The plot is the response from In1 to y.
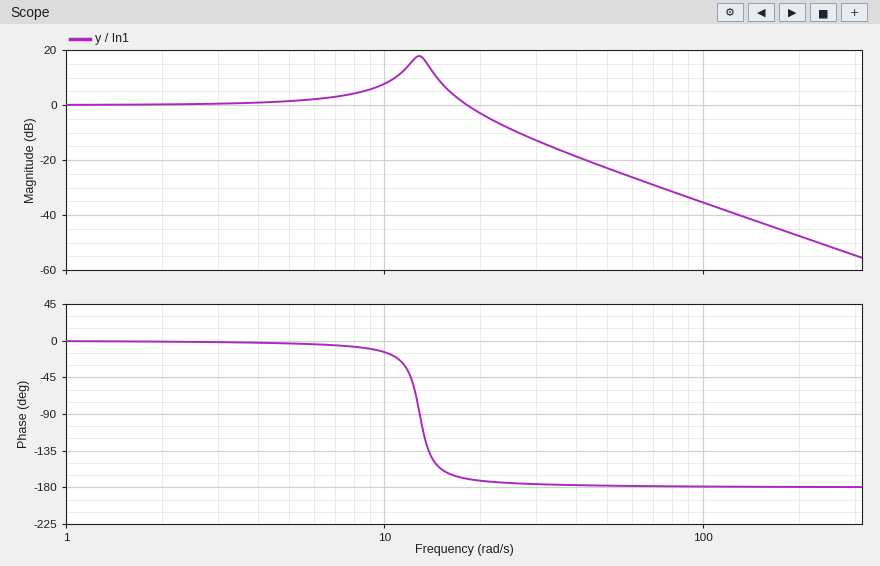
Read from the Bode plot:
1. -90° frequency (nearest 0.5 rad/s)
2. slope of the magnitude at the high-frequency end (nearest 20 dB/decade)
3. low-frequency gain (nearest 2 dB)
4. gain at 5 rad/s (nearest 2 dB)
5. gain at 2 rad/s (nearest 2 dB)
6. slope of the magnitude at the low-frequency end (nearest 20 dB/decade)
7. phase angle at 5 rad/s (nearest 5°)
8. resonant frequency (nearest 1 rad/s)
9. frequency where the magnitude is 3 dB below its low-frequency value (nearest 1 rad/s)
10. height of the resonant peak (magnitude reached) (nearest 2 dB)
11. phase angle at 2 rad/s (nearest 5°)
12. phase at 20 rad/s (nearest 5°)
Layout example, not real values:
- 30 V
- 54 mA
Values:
- 13.0 rad/s
- -40 dB/decade
- 0 dB
- 2 dB
- 0 dB
- 0 dB/decade
- -5°
- 13 rad/s
- 20 rad/s
- 18 dB
- 0°
- -170°
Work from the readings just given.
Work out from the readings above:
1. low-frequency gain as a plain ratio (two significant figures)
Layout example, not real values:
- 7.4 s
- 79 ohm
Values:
- 1.0
